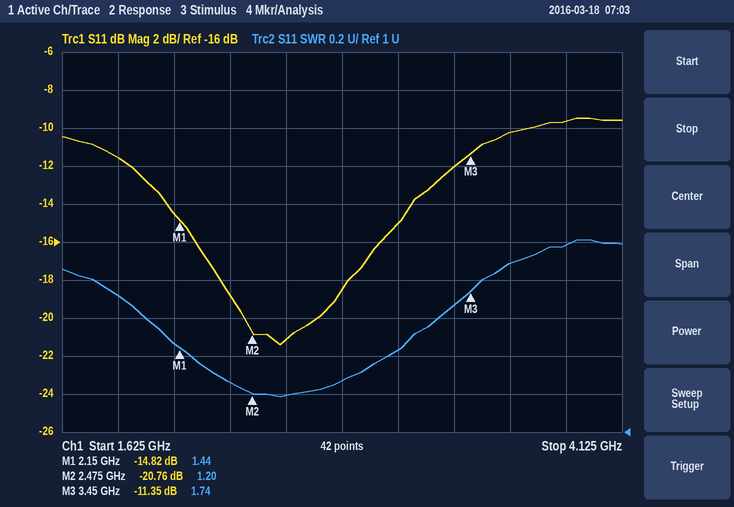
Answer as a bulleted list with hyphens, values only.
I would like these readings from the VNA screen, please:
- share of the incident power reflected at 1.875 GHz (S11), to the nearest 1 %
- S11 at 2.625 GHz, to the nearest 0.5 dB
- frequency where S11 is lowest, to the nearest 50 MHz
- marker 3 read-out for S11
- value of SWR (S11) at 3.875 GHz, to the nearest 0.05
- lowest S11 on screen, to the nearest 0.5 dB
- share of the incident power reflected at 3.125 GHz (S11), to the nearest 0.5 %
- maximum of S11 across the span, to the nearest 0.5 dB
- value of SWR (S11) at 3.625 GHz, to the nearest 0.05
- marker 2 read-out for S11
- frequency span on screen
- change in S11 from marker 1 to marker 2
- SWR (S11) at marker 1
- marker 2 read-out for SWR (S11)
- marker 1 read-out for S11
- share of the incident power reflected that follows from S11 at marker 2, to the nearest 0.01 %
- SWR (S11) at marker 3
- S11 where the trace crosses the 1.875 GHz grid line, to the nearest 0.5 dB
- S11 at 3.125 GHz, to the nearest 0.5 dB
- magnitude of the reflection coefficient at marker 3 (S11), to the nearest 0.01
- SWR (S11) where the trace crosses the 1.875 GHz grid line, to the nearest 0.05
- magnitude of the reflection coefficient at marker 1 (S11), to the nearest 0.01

- 7 %
- -21.0 dB
- 2.60 GHz
- -11.35 dB
- 2.00
- -21.5 dB
- 3.0 %
- -9.5 dB
- 1.90
- -20.76 dB
- 2.5 GHz
- -5.94 dB
- 1.44
- 1.20
- -14.82 dB
- 0.84 %
- 1.74
- -11.5 dB
- -15.0 dB
- 0.27
- 1.70
- 0.18
